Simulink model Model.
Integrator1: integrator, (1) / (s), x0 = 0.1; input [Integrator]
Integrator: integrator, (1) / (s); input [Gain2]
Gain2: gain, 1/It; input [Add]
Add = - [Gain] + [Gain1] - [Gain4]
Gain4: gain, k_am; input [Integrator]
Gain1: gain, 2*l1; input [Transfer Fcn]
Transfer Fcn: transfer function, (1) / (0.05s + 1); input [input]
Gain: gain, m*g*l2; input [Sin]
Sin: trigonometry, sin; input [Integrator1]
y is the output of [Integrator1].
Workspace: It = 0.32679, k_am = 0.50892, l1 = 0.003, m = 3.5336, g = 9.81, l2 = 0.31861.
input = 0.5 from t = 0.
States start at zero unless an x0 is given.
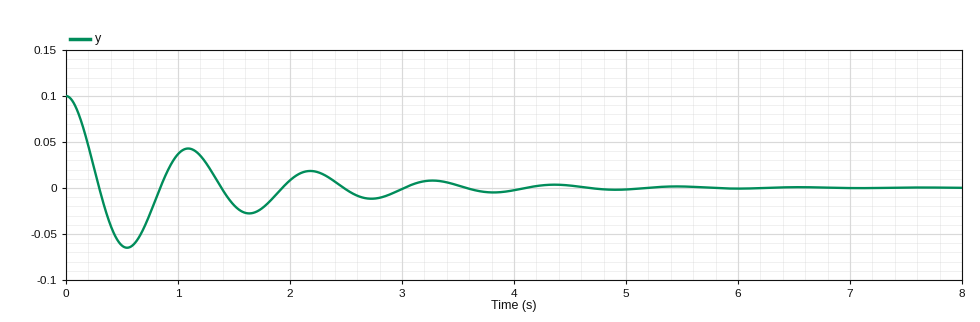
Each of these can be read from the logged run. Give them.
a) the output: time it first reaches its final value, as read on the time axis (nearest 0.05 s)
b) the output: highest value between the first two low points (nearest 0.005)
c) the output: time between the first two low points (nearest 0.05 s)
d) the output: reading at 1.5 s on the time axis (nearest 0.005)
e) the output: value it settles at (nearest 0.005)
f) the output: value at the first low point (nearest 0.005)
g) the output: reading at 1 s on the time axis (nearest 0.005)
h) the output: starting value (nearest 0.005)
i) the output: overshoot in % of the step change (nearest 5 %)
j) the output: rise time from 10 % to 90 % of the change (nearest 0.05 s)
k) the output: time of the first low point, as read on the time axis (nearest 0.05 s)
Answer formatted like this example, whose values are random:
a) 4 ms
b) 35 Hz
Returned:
a) 0.30 s
b) 0.045
c) 1.10 s
d) -0.020
e) 0.000
f) -0.065
g) 0.035
h) 0.100
i) 65 %
j) 0.20 s
k) 0.55 s
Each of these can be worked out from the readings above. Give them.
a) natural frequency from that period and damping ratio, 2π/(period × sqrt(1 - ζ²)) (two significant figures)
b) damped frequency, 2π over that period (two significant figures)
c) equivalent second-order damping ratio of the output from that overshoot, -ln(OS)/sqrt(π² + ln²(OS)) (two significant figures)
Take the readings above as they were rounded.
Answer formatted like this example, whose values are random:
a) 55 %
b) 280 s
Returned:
a) 5.8 rad/s
b) 5.7 rad/s
c) 0.14
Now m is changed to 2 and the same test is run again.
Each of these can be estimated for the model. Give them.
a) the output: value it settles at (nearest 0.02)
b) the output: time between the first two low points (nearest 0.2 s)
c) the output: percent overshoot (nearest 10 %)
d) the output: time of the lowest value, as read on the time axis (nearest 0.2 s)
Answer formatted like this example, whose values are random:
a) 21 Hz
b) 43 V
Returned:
a) 0.00
b) 1.4 s
c) 60 %
d) 0.8 s
